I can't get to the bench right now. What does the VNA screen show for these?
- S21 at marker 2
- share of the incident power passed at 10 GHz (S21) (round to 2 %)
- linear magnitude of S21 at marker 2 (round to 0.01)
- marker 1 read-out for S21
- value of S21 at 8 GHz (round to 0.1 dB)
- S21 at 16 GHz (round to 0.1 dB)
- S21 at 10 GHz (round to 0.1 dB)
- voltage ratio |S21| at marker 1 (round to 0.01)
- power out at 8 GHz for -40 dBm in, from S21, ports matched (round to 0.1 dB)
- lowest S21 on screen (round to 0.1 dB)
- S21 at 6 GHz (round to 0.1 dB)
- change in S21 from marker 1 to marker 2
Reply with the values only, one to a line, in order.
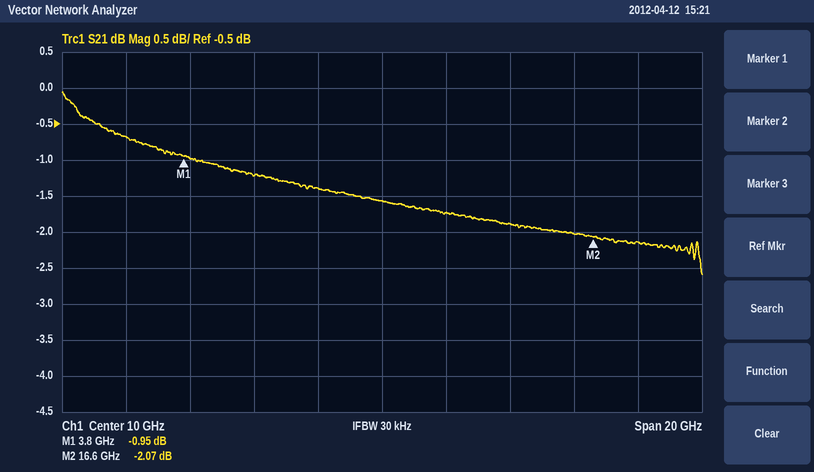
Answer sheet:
-2.07 dB
70 %
0.79
-0.95 dB
-1.4 dB
-2.0 dB
-1.6 dB
0.90
-41.4 dBm
-2.6 dB
-1.2 dB
-1.12 dB
